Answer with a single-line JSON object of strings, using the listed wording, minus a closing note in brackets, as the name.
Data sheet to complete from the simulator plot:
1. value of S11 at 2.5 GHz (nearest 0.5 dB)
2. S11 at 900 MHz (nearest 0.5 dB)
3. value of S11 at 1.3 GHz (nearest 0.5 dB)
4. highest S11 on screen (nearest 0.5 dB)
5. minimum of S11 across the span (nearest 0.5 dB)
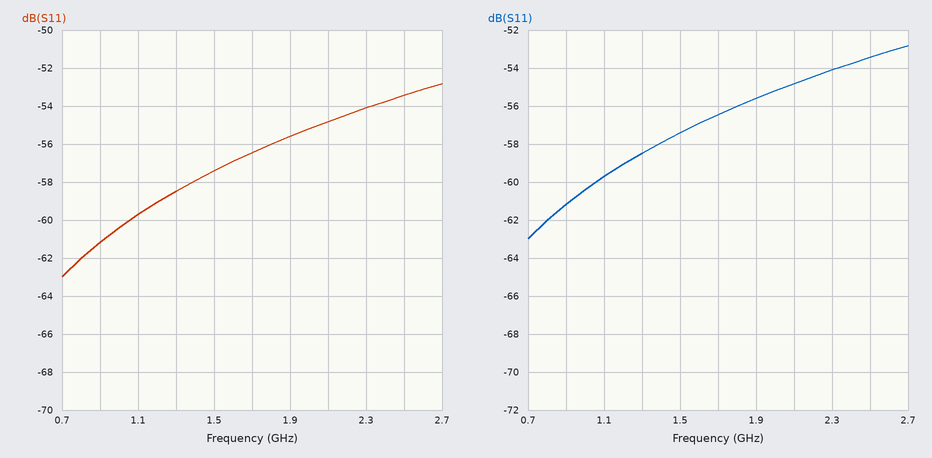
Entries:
{"value of S11 at 2.5 GHz": "-53.5 dB", "S11 at 900 MHz": "-61.0 dB", "value of S11 at 1.3 GHz": "-58.5 dB", "highest S11 on screen": "-53.0 dB", "minimum of S11 across the span": "-63.0 dB"}
